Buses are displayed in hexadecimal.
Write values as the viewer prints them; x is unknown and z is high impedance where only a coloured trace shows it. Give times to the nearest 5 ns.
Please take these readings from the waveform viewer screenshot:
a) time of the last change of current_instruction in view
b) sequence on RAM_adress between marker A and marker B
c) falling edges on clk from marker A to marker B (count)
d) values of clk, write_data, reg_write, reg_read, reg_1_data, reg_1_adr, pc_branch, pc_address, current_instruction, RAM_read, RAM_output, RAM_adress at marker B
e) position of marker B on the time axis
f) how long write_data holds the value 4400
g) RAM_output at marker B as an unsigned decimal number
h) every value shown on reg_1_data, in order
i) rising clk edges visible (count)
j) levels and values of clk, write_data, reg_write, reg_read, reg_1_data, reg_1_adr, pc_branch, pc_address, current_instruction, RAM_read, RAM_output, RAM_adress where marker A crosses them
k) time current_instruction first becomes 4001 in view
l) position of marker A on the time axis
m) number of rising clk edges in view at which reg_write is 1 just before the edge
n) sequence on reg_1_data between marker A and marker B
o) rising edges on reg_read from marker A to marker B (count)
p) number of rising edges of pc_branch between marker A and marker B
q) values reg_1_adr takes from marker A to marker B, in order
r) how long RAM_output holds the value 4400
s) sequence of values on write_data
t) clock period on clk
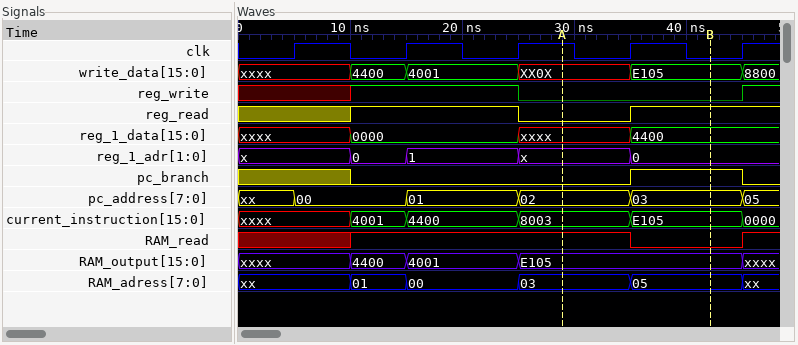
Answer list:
45 ns
03, 05
2
clk=0, write_data=E105, reg_write=0, reg_read=1, reg_1_data=4400, reg_1_adr=0, pc_branch=1, pc_address=03, current_instruction=E105, RAM_read=0, RAM_output=E105, RAM_adress=05
40 ns
5 ns
57605
xxxx, 0000, xxxx, 4400
5
clk=1, write_data=XX0X, reg_write=0, reg_read=0, reg_1_data=xxxx, reg_1_adr=x, pc_branch=0, pc_address=02, current_instruction=8003, RAM_read=1, RAM_output=E105, RAM_adress=03
10 ns
30 ns
2
xxxx, 4400
1
1
x, 0
5 ns
xxxx, 4400, 4001, XX0X, E105, 8800
10 ns
